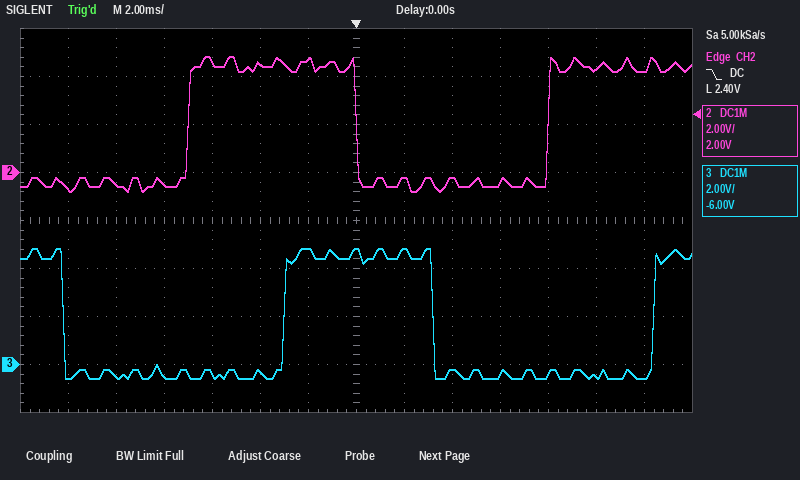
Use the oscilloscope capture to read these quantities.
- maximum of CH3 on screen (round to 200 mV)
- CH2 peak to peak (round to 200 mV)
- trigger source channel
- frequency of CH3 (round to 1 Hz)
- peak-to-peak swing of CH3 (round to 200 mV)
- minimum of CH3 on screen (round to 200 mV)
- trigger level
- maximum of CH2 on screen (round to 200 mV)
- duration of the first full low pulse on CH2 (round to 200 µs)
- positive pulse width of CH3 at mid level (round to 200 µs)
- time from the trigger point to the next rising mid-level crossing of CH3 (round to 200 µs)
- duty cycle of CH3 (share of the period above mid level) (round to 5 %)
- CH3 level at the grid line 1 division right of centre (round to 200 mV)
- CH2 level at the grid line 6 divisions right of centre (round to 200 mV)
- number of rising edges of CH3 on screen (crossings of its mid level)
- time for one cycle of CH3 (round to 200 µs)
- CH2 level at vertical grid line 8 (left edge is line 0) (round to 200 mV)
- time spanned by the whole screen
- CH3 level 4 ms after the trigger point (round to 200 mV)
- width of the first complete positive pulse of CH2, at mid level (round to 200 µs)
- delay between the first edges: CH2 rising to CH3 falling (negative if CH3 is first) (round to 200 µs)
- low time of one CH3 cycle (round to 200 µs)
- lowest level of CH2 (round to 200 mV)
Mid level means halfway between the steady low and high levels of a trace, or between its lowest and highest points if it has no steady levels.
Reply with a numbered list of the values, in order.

1. 4.8 V
2. 5.6 V
3. CH2
4. 65 Hz
5. 5.4 V
6. -600 mV
7. 2.40 V
8. 4.8 V
9. 8.0 ms
10. 6.2 ms
11. 12.4 ms
12. 40 %
13. 4.8 V
14. 4.2 V
15. 2
16. 15.4 ms
17. -200 mV
18. 28 ms
19. -200 mV
20. 7.0 ms
21. -5.2 ms
22. 9.2 ms
23. -800 mV
